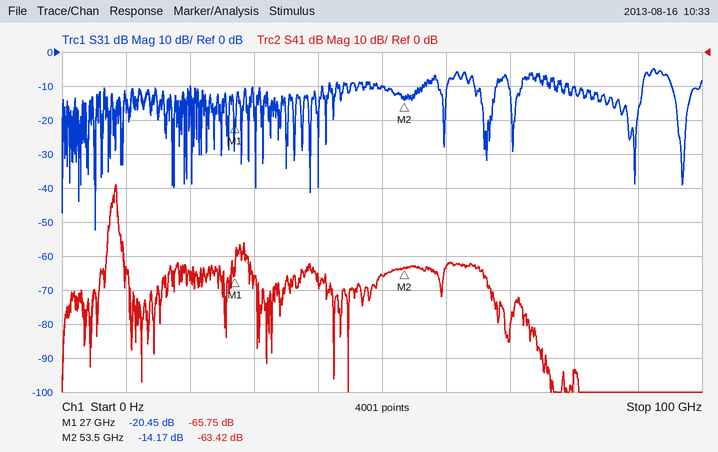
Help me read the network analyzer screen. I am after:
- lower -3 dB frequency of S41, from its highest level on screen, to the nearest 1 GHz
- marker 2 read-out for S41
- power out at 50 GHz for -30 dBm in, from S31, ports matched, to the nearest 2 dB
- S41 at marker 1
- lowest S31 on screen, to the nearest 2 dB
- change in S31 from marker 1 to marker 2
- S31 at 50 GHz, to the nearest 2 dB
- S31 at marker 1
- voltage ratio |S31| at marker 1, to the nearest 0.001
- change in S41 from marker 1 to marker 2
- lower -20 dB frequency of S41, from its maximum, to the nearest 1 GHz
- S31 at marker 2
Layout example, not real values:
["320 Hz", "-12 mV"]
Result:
["8 GHz", "-63.42 dB", "-40 dBm", "-65.75 dB", "-52 dB", "6.28 dB", "-10 dB", "-20.45 dB", "0.095", "2.33 dB", "7 GHz", "-14.17 dB"]
